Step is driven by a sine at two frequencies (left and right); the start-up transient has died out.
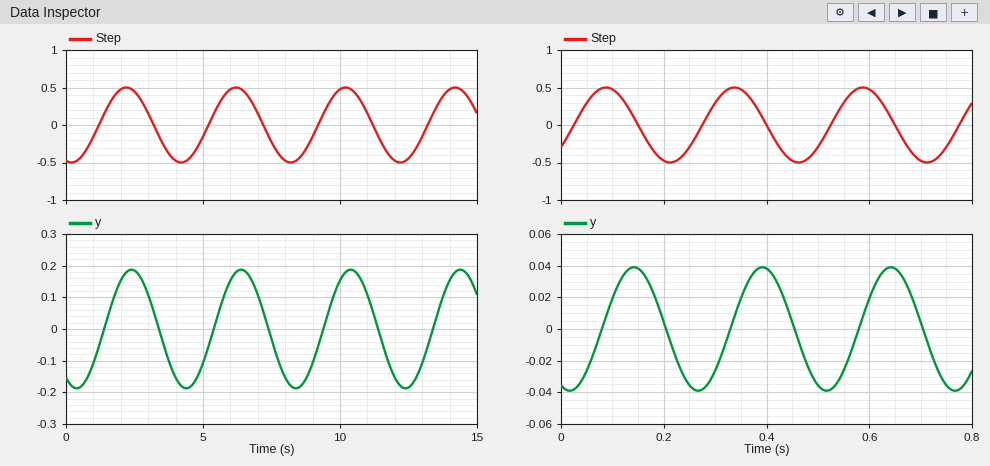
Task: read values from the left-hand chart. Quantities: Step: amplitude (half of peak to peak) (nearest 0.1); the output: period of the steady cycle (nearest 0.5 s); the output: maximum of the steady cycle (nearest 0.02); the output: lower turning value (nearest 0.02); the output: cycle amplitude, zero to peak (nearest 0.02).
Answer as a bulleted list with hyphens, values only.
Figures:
- 0.5
- 4.0 s
- 0.18
- -0.18
- 0.18
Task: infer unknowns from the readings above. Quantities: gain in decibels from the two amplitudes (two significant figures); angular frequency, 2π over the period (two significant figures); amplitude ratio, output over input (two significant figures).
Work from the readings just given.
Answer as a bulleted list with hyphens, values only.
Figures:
- -8.9 dB
- 1.6 rad/s
- 0.36
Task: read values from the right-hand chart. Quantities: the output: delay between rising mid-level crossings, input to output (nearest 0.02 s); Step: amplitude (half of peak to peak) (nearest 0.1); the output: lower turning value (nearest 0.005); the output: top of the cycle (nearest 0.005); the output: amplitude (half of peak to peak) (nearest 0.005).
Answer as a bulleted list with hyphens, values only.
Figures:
- 0.06 s
- 0.5
- -0.040
- 0.040
- 0.040
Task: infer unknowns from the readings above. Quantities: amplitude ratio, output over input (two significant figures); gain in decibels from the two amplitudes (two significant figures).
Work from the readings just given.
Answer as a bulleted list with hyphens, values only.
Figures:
- 0.080
- -22 dB
